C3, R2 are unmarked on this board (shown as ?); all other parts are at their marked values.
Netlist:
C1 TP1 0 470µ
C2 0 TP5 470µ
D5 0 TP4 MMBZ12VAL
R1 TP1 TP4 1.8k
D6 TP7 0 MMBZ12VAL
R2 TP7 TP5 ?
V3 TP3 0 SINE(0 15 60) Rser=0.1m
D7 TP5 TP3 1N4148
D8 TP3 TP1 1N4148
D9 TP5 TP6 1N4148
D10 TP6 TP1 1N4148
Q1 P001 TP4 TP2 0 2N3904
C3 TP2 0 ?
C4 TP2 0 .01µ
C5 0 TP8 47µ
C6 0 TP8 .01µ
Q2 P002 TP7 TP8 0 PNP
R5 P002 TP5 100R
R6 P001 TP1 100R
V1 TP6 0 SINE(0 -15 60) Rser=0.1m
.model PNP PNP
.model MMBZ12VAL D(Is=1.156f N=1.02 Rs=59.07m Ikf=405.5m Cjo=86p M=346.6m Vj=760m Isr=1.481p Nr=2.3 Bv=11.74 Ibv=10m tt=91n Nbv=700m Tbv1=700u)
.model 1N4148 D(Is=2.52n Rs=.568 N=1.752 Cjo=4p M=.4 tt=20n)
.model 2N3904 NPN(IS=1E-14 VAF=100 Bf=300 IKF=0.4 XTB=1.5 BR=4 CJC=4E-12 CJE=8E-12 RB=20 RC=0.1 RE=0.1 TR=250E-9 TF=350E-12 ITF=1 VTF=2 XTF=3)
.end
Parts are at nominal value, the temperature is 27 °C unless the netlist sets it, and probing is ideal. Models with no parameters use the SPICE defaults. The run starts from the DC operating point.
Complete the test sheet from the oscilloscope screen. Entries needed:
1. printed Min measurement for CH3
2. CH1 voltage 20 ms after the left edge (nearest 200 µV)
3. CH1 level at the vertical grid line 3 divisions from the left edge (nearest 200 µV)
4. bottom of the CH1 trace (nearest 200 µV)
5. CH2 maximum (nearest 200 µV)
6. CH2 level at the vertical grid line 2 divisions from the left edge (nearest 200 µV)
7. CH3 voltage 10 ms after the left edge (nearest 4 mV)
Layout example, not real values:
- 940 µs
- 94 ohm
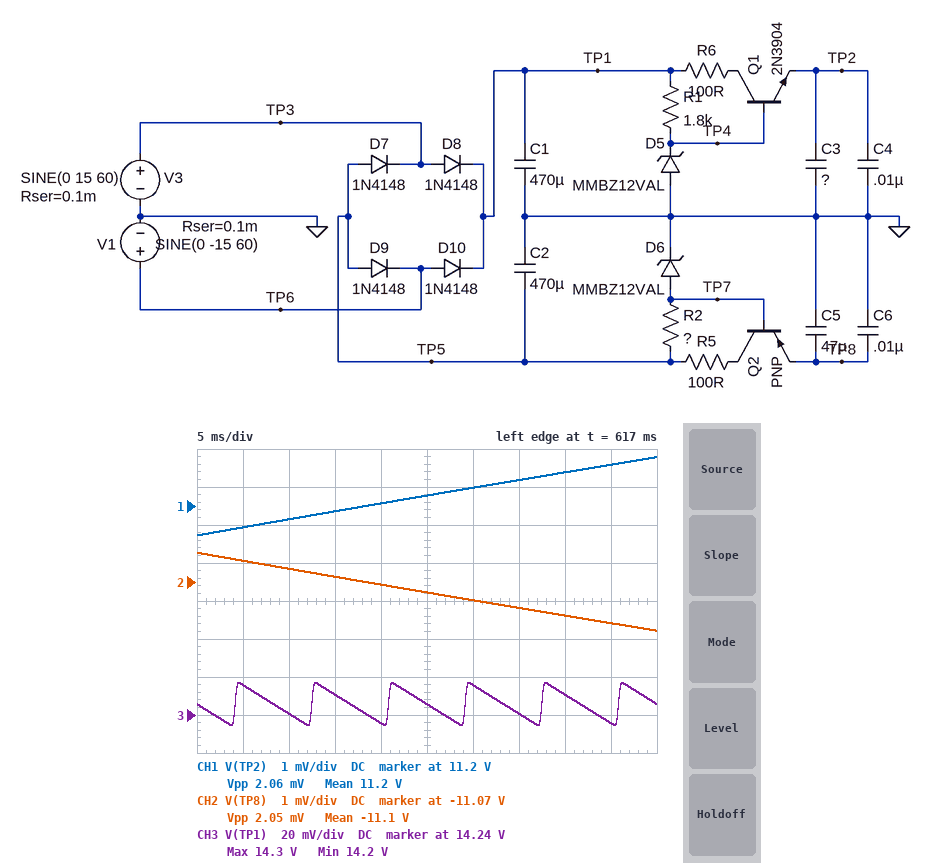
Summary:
- 14.2 V
- 11.2020 V
- 11.2018 V
- 11.2012 V
- -11.0712 V
- -11.0716 V
- 14.240 V
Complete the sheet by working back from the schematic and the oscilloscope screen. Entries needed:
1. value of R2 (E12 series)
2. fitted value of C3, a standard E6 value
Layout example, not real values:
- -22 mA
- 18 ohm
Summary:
- 5.6 kΩ
- 68 µF
